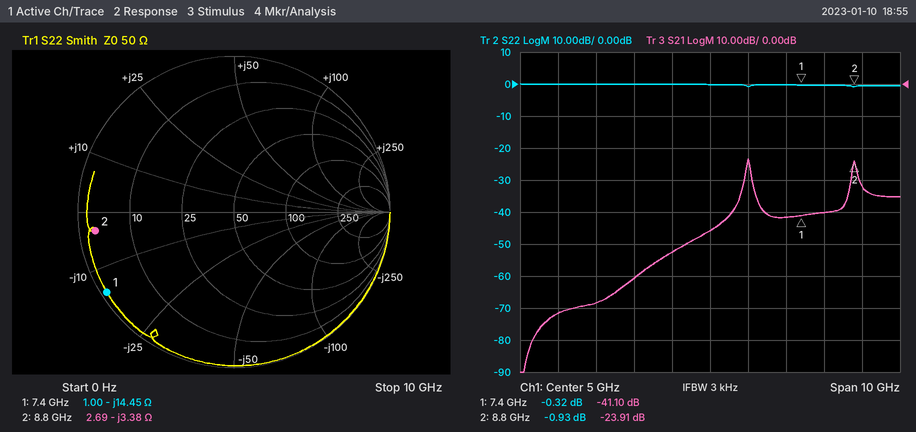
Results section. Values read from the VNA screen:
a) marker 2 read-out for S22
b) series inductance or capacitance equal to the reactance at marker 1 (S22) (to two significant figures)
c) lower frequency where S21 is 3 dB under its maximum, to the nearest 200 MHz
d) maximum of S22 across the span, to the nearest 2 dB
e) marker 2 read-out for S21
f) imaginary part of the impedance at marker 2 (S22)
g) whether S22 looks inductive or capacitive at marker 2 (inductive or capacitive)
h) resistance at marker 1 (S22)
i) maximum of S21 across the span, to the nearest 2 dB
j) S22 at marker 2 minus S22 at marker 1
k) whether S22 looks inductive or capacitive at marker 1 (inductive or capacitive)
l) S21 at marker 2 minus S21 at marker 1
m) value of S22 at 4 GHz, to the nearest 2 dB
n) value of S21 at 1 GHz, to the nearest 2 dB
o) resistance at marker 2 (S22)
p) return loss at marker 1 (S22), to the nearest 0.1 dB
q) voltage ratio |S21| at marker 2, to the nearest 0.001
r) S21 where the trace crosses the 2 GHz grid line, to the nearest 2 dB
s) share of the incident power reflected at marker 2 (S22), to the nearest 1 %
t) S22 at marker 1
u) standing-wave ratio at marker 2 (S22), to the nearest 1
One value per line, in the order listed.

-0.93 dB
1.5 pF
6.0 GHz
0 dB
-23.91 dB
-3.38 Ω
capacitive
1.00 Ω
-24 dB
-0.61 dB
capacitive
17.19 dB
0 dB
-72 dB
2.69 Ω
0.3 dB
0.064
-68 dB
81 %
-0.32 dB
19
